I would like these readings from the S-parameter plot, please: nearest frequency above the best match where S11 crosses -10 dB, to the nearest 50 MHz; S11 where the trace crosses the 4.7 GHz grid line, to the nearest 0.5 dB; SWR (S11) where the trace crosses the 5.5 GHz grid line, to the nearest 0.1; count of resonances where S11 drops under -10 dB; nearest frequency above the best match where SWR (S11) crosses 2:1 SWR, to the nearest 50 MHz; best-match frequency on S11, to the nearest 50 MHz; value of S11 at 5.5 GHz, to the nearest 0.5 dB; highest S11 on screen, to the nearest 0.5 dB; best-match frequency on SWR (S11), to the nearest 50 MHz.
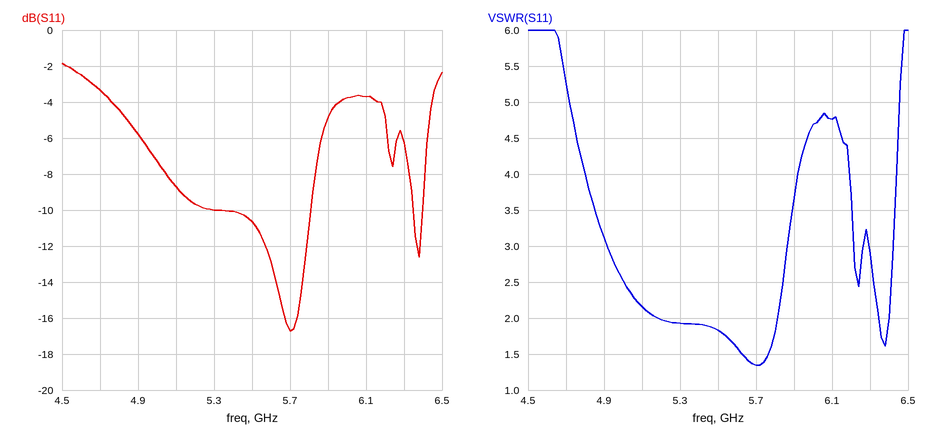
5.80 GHz
-3.5 dB
1.8
2
5.80 GHz
5.70 GHz
-10.5 dB
-2.0 dB
5.70 GHz
